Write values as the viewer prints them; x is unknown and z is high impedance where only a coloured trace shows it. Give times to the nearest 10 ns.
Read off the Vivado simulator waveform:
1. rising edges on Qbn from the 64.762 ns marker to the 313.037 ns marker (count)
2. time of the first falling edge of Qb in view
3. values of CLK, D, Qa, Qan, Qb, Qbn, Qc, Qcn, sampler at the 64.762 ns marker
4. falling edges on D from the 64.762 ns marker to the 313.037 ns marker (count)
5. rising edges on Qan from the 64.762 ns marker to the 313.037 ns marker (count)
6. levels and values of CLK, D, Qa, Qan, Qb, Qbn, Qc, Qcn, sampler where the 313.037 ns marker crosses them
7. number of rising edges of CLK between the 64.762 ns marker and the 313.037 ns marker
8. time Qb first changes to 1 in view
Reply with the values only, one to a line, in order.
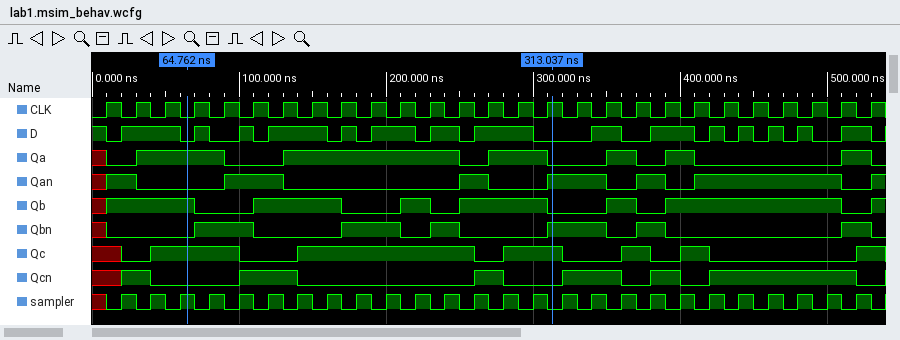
4
70 ns
CLK=0, D=0, Qa=1, Qan=0, Qb=1, Qbn=0, Qc=1, Qcn=0, sampler=1
7
3
CLK=1, D=0, Qa=0, Qan=1, Qb=0, Qbn=1, Qc=1, Qcn=0, sampler=0
13
10 ns
